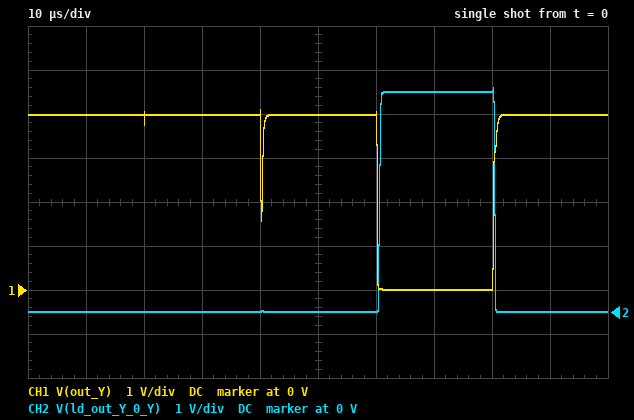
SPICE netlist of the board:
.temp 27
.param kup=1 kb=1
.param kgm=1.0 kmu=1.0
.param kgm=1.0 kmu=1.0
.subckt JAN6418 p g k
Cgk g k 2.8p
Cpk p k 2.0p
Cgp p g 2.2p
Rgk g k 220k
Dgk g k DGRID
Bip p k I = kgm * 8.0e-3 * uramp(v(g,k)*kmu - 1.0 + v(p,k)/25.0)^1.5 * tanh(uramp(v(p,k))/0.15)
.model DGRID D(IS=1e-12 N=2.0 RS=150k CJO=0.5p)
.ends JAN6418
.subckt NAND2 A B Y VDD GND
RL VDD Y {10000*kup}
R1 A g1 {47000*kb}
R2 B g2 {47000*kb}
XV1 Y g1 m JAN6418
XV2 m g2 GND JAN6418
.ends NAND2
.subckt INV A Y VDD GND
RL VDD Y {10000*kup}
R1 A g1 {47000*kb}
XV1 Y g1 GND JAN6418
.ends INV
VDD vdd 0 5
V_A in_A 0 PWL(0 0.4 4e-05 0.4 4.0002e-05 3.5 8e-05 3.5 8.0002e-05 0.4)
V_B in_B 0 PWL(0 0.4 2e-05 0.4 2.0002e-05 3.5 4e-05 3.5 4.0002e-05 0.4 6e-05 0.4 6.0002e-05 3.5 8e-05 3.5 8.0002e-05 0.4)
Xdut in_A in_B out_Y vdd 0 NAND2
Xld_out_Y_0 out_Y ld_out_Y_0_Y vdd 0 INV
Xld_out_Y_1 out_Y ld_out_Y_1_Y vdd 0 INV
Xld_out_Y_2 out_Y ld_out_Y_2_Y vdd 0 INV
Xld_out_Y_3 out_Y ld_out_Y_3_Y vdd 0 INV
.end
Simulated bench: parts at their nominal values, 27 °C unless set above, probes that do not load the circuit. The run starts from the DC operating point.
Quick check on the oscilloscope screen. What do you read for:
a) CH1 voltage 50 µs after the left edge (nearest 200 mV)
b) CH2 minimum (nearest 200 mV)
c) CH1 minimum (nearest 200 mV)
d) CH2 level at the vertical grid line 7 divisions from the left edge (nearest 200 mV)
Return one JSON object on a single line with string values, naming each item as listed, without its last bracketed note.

{"CH1 voltage 50 µs after the left edge": "4.0 V", "CH2 minimum": "0 V", "CH1 minimum": "0 V", "CH2 level at the vertical grid line 7 divisions from the left edge": "5.0 V"}
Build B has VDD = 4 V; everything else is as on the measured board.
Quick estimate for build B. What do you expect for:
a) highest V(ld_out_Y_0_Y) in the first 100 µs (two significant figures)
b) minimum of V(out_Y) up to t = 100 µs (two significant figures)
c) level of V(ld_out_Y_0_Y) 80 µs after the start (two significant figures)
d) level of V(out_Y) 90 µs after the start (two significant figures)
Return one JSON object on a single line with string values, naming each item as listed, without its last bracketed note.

{"highest V(ld_out_Y_0_Y) in the first 100 µs": "4.1 V", "minimum of V(out_Y) up to t = 100 µs": "7.5 mV", "level of V(ld_out_Y_0_Y) 80 µs after the start": "4.0 V", "level of V(out_Y) 90 µs after the start": "3.2 V"}
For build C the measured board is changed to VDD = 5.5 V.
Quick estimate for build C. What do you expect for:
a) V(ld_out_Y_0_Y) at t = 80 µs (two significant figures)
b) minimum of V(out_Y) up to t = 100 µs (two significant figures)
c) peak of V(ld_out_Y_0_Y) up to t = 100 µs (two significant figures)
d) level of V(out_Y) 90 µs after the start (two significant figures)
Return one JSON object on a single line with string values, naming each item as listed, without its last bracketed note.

{"V(ld_out_Y_0_Y) at t = 80 µs": "5.5 V", "minimum of V(out_Y) up to t = 100 µs": "11 mV", "peak of V(ld_out_Y_0_Y) up to t = 100 µs": "5.6 V", "level of V(out_Y) 90 µs after the start": "4.4 V"}
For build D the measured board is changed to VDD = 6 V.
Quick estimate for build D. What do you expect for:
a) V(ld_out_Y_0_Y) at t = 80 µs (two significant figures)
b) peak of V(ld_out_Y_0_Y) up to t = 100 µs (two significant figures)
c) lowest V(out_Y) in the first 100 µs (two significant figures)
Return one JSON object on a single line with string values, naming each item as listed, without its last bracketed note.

{"V(ld_out_Y_0_Y) at t = 80 µs": "6.0 V", "peak of V(ld_out_Y_0_Y) up to t = 100 µs": "6.1 V", "lowest V(out_Y) in the first 100 µs": "12 mV"}
